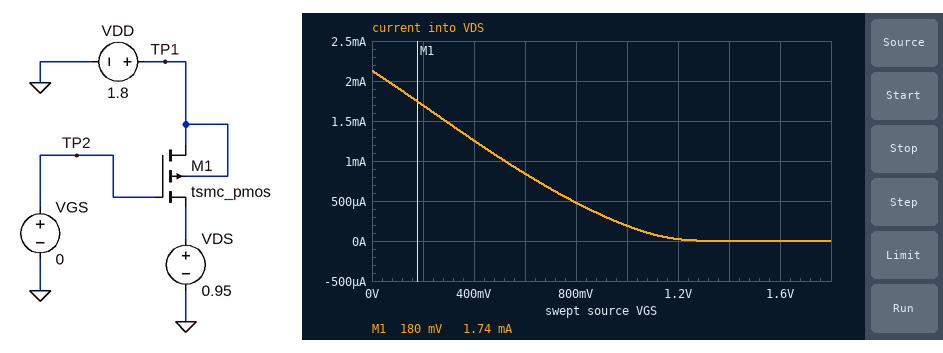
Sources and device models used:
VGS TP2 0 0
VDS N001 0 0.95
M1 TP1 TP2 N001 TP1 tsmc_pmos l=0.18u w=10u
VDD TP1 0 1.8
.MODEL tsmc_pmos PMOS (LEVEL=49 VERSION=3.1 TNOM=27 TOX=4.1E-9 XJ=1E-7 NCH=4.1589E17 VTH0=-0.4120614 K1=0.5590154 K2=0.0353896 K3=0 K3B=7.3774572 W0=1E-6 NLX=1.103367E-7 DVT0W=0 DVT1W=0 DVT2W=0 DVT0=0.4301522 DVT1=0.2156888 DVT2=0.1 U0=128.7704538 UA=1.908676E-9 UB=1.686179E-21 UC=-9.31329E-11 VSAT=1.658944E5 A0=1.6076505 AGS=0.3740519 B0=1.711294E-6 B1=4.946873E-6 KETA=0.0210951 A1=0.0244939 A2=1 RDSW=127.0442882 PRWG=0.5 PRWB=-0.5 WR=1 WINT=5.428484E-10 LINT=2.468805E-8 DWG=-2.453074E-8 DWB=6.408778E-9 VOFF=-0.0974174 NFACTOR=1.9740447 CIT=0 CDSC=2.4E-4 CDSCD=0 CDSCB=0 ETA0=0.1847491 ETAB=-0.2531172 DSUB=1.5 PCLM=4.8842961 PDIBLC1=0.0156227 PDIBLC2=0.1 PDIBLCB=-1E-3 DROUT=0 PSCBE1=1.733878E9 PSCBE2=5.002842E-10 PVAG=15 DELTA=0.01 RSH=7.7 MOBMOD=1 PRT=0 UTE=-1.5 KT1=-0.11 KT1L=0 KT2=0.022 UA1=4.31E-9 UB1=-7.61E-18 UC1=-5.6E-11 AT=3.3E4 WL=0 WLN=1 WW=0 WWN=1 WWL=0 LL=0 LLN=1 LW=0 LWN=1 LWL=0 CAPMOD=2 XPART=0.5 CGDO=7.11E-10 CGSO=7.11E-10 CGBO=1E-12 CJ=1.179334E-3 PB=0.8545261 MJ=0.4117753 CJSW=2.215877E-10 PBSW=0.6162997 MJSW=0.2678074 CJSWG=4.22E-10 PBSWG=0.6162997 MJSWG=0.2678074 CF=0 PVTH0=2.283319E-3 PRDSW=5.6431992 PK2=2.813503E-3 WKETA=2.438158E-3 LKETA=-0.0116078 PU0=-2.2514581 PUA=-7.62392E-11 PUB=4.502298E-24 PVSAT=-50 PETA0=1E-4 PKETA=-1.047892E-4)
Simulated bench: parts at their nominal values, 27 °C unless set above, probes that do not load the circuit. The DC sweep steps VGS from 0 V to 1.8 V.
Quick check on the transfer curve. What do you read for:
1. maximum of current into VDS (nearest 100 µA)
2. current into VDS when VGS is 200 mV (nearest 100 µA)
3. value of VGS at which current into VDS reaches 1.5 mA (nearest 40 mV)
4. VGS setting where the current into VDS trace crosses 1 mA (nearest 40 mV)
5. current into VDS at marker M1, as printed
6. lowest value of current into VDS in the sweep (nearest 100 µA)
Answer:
2.1 mA
1.7 mA
280 mV
520 mV
1.74 mA
0 A
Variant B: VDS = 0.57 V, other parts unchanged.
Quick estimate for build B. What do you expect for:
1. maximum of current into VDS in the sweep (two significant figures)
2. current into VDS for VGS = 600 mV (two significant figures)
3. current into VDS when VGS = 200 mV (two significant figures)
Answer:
2.3 mA
890 µA
1.8 mA
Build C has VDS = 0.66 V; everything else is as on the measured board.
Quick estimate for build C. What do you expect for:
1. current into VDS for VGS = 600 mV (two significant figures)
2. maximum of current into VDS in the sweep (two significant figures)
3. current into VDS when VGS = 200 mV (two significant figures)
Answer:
880 µA
2.3 mA
1.8 mA
